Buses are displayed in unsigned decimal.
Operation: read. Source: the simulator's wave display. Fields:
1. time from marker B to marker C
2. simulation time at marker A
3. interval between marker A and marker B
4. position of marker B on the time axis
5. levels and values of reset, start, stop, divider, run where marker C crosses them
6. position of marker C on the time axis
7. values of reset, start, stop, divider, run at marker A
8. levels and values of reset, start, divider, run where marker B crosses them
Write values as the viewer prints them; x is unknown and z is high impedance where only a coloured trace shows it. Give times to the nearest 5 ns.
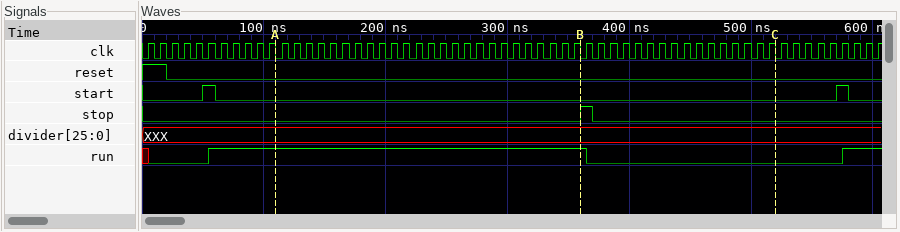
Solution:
160 ns
110 ns
250 ns
360 ns
reset=0, start=0, stop=0, divider=XXX, run=0
520 ns
reset=0, start=0, stop=0, divider=XXX, run=1
reset=0, start=0, divider=XXX, run=1
